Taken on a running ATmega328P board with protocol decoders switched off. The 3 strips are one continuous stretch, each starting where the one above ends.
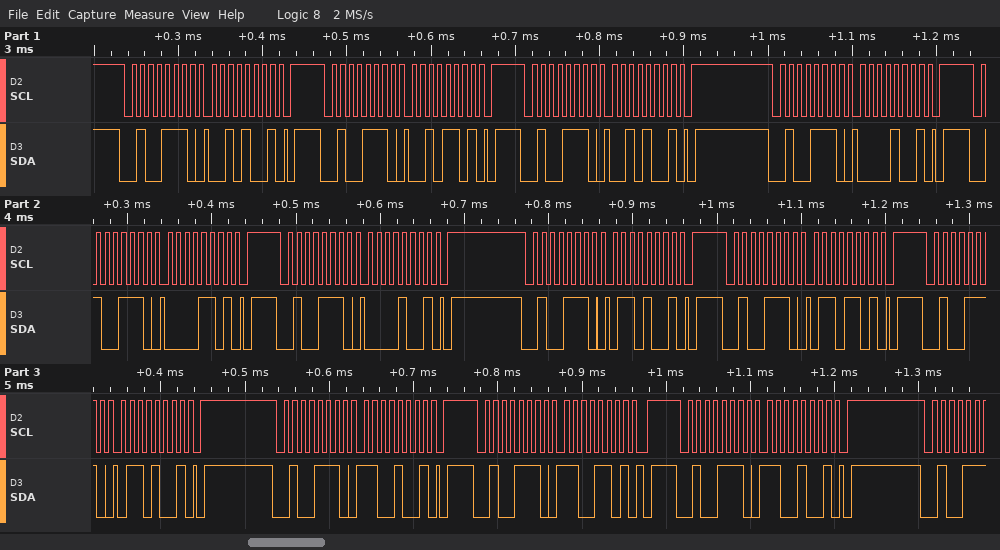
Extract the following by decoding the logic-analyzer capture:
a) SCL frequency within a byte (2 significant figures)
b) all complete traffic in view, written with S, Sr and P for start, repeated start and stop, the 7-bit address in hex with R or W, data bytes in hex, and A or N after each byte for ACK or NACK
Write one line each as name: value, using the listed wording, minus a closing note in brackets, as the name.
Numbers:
SCL frequency within a byte: 100 kHz
all complete traffic in view, written with S, Sr and P for start, repeated start and stop, the 7-bit address in hex with R or W, data bytes in hex, and A or N after each byte for ACK or NACK: S 27W A 29 A P S 27W A 2D A P S 27W A 29 A P S 27W A 09 A P S 27W A 0D A P S 27W A 09 A P S 27W A 69 A P S 27W A 6D A P S 27W A 69 A P S 27W A C9 A P S 27W A CD A P S 27W A C9 A P
